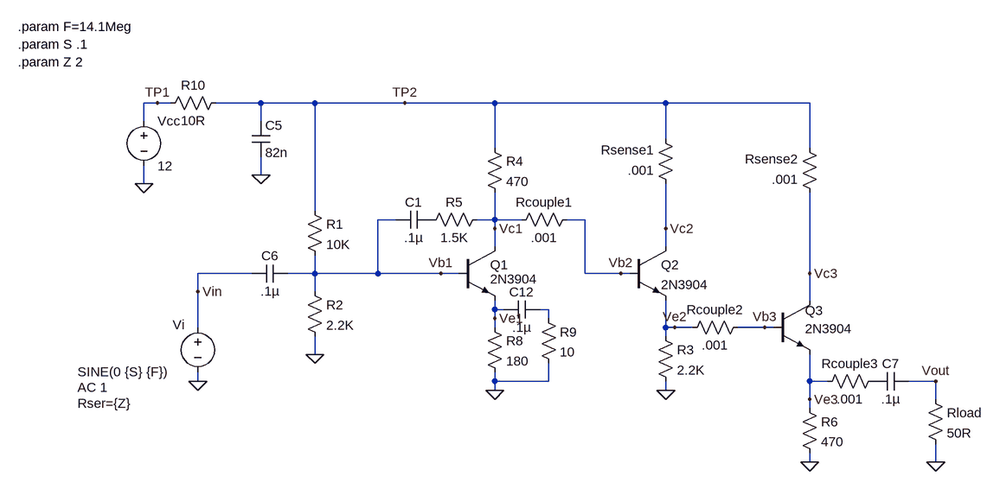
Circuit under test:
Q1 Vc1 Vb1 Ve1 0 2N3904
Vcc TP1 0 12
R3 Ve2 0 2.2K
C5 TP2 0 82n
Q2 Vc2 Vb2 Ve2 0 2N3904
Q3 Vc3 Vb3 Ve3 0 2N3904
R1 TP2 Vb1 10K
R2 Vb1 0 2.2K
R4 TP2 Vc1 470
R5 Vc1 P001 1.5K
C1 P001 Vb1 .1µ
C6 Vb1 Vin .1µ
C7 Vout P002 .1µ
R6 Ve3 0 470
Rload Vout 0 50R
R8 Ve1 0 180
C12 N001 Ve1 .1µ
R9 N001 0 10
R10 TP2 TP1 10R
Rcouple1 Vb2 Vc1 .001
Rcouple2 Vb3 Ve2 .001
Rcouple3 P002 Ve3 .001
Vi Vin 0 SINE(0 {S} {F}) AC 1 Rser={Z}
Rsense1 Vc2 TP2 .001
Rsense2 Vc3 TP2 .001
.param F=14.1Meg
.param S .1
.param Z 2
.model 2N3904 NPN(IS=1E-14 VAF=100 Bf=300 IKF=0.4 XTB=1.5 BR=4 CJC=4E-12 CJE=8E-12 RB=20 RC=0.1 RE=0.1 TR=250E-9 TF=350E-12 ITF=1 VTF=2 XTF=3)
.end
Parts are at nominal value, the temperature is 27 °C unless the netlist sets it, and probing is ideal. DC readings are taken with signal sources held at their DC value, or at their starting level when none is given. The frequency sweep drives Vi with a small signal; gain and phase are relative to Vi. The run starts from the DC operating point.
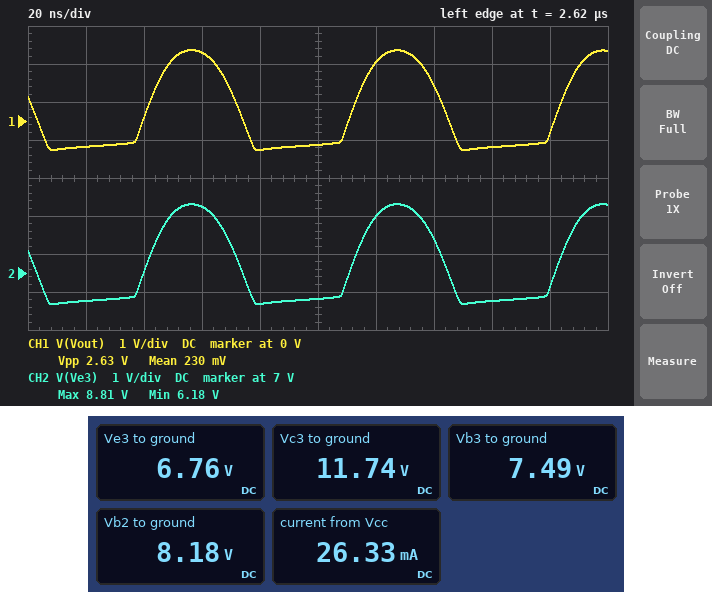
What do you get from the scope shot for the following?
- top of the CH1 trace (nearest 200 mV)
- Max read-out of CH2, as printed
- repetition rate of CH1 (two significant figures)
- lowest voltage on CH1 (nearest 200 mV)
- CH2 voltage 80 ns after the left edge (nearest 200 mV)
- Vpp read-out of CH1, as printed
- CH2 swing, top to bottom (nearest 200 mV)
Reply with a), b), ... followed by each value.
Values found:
a) 1.8 V
b) 8.81 V
c) 14 MHz
d) -800 mV
e) 6.2 V
f) 2.63 V
g) 2.6 V
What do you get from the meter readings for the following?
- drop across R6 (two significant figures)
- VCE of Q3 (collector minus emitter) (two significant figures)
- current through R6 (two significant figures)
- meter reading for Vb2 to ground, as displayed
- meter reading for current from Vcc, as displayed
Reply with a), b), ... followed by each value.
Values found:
a) 6.8 V
b) 5.0 V
c) 14 mA
d) 8.18 V
e) 26.33 mA
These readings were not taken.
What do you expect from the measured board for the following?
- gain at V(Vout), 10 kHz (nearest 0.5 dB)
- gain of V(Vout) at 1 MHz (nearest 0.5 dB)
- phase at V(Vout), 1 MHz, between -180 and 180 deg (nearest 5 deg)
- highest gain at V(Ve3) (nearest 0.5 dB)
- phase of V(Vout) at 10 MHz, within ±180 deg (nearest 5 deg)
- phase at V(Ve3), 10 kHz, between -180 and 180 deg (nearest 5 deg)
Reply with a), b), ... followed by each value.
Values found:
a) -4.0 dB
b) 27.5 dB
c) -170 deg
d) 28.0 dB
e) 165 deg
f) -120 deg
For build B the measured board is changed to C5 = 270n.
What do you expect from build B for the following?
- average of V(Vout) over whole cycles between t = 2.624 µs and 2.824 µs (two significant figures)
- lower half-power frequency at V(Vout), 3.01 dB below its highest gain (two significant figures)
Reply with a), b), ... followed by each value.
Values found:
a) 310 mV
b) 150 kHz
